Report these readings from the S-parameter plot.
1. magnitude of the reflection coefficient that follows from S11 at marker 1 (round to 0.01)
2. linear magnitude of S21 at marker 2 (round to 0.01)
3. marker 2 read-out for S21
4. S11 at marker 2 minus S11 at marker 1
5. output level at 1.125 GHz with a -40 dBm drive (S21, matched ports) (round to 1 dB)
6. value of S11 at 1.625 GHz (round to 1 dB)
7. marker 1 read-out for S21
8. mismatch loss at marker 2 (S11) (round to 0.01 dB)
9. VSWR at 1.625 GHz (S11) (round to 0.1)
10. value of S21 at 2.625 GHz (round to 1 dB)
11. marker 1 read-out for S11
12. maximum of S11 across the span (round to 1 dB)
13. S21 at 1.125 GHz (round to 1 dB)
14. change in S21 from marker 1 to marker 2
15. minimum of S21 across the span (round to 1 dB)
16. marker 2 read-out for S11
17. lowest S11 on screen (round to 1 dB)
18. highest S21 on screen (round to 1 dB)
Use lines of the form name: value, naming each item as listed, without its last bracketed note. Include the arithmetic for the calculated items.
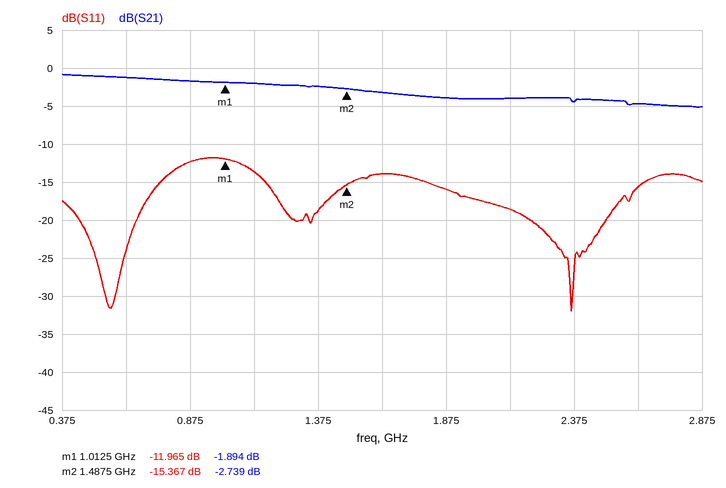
magnitude of the reflection coefficient that follows from S11 at marker 1: 10^(-11.965/20) ≈ 0.25
linear magnitude of S21 at marker 2: 10^(-2.739/20) ≈ 0.73
marker 2 read-out for S21: -2.739 dB
S11 at marker 2 minus S11 at marker 1: -15.367 − (-11.965) = -3.402 dB
output level at 1.125 GHz with a -40 dBm drive (S21, matched ports): -40 dBm + (-2 dB) = -42 dBm
value of S11 at 1.625 GHz: -14 dB
marker 1 read-out for S21: -1.894 dB
mismatch loss at marker 2 (S11): −10 log10(1 − 10^(-15.367/10)) ≈ 0.13 dB
VSWR at 1.625 GHz (S11): |Γ| = 10^(-14/20) = 0.1995; VSWR = (1 + 0.1995)/(1 − 0.1995) ≈ 1.5
value of S21 at 2.625 GHz: -5 dB
marker 1 read-out for S11: -11.965 dB
maximum of S11 across the span: -12 dB
S21 at 1.125 GHz: -2 dB
change in S21 from marker 1 to marker 2: -2.739 − (-1.894) = -0.845 dB
minimum of S21 across the span: -5 dB
marker 2 read-out for S11: -15.367 dB
lowest S11 on screen: -32 dB
highest S21 on screen: -1 dB
